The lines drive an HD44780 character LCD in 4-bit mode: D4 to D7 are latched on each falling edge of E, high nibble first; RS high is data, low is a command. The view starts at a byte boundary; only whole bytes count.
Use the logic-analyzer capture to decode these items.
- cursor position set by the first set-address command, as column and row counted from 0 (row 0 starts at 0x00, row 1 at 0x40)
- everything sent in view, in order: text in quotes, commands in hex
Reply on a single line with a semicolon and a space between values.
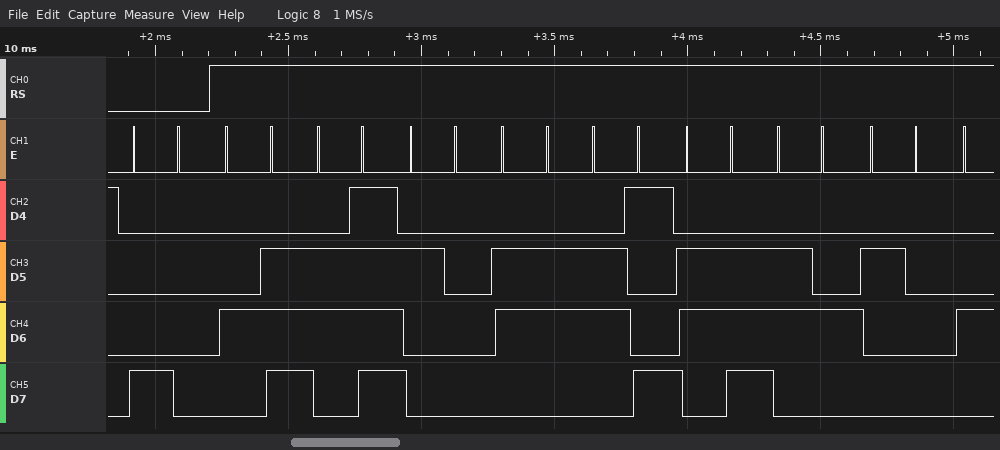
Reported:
column 0, row 0; 0x80 "No find "
